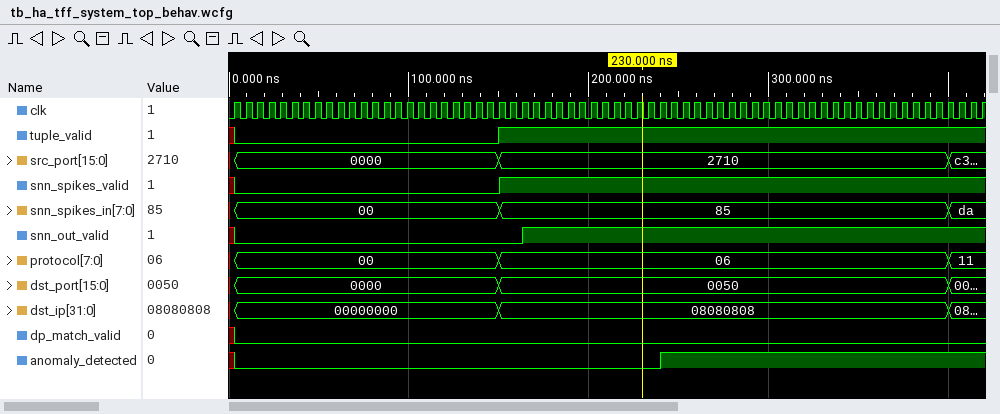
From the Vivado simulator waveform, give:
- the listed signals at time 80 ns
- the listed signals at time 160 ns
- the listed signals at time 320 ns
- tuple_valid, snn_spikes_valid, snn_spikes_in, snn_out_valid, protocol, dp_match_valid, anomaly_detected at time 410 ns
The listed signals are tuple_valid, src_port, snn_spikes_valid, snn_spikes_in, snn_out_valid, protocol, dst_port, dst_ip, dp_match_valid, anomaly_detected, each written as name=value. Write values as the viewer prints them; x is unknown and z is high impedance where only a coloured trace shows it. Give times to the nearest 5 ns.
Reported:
tuple_valid=0, src_port=0000, snn_spikes_valid=0, snn_spikes_in=00, snn_out_valid=0, protocol=00, dst_port=0000, dst_ip=00000000, dp_match_valid=0, anomaly_detected=0
tuple_valid=1, src_port=2710, snn_spikes_valid=1, snn_spikes_in=85, snn_out_valid=0, protocol=06, dst_port=0050, dst_ip=08080808, dp_match_valid=0, anomaly_detected=0
tuple_valid=1, src_port=2710, snn_spikes_valid=1, snn_spikes_in=85, snn_out_valid=1, protocol=06, dst_port=0050, dst_ip=08080808, dp_match_valid=0, anomaly_detected=1
tuple_valid=1, snn_spikes_valid=1, snn_spikes_in=da, snn_out_valid=1, protocol=11, dp_match_valid=0, anomaly_detected=1
